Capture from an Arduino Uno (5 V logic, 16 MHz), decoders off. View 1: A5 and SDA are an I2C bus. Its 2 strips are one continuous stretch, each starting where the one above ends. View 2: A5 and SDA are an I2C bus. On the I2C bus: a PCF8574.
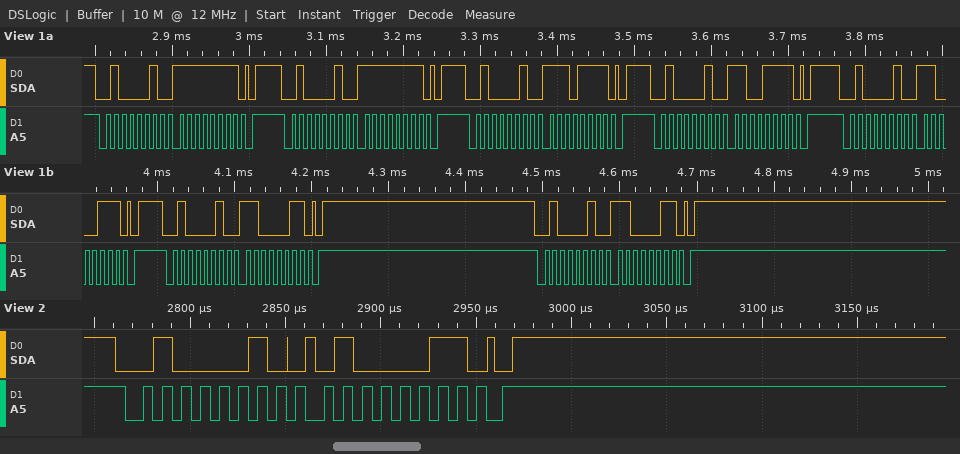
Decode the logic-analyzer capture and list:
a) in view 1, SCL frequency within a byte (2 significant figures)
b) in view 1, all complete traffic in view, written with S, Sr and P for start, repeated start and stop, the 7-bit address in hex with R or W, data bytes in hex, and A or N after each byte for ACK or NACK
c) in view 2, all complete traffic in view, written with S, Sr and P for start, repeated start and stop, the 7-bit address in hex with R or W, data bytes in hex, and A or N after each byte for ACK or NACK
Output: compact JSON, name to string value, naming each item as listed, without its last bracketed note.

{"in view 1, SCL frequency within a byte": "100 kHz", "in view 1, all complete traffic in view, written with S, Sr and P for start, repeated start and stop, the 7-bit address in hex with R or W, data bytes in hex, and A or N after each byte for ACK or NACK": "S 21W A FF A P S 21W A FF A P S 21W A EF A P S 21W A CF A P S 21W A C7 A P S 21W A C3 A P S 21W A C3 A P", "in view 2, all complete traffic in view, written with S, Sr and P for start, repeated start and stop, the 7-bit address in hex with R or W, data bytes in hex, and A or N after each byte for ACK or NACK": "S 21W A 43 A P"}
